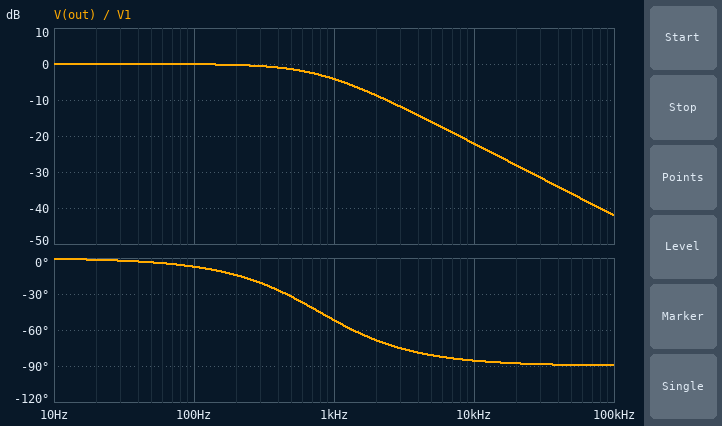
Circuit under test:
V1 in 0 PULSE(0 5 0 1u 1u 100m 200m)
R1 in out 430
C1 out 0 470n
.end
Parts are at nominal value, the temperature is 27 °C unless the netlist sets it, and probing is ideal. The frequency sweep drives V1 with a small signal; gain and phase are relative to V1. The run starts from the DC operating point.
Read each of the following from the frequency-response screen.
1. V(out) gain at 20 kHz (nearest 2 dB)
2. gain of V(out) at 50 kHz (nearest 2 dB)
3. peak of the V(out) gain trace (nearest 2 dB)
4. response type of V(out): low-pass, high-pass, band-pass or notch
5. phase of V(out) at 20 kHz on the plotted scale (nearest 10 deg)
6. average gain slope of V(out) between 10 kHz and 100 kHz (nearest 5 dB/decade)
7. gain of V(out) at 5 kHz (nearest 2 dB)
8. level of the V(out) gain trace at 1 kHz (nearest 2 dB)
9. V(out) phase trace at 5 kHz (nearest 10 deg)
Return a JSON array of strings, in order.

["-28 dB", "-36 dB", "0 dB", "low-pass", "-90 deg", "-20 dB/decade", "-16 dB", "-4 dB", "-80 deg"]
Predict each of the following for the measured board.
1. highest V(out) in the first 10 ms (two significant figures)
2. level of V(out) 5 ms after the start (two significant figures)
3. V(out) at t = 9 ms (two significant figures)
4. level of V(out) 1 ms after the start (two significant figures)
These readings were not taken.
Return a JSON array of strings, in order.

["5.0 V", "5.0 V", "5.0 V", "5.0 V"]
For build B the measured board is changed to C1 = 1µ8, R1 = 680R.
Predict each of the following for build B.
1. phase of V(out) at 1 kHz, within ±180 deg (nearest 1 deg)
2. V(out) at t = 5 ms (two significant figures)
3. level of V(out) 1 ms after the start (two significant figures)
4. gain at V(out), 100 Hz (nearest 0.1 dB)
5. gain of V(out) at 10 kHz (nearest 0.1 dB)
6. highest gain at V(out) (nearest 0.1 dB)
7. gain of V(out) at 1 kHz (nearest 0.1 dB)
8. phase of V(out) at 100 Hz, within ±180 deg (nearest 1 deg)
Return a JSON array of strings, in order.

["-83 deg", "4.9 V", "2.8 V", "-2.0 dB", "-37.7 dB", "0 dB", "-17.8 dB", "-38 deg"]
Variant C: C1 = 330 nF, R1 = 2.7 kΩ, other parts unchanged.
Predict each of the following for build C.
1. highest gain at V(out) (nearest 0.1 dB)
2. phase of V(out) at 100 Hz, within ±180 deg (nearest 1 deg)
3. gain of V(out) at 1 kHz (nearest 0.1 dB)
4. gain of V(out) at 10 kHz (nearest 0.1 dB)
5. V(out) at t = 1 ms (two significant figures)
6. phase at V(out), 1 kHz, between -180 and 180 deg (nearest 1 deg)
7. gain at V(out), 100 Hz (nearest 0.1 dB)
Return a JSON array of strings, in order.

["0 dB", "-29 deg", "-15.1 dB", "-35.0 dB", "3.4 V", "-80 deg", "-1.2 dB"]
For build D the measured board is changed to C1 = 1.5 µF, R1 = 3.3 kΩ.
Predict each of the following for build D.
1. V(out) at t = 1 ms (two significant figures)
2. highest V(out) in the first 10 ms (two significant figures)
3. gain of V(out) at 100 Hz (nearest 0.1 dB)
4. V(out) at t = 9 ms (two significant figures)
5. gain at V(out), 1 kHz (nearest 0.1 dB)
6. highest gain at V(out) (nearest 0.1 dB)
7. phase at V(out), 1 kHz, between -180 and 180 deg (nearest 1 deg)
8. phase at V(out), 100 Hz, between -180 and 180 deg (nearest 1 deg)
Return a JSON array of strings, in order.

["910 mV", "4.3 V", "-10.3 dB", "4.2 V", "-29.9 dB", "0 dB", "-88 deg", "-72 deg"]
